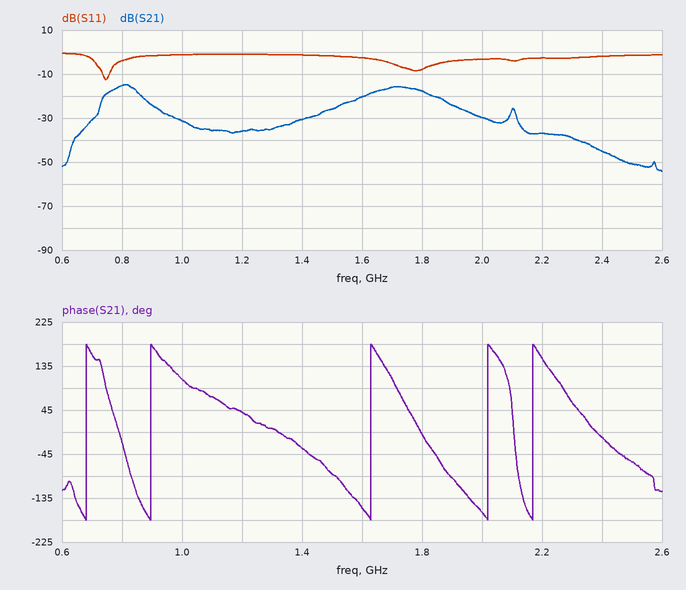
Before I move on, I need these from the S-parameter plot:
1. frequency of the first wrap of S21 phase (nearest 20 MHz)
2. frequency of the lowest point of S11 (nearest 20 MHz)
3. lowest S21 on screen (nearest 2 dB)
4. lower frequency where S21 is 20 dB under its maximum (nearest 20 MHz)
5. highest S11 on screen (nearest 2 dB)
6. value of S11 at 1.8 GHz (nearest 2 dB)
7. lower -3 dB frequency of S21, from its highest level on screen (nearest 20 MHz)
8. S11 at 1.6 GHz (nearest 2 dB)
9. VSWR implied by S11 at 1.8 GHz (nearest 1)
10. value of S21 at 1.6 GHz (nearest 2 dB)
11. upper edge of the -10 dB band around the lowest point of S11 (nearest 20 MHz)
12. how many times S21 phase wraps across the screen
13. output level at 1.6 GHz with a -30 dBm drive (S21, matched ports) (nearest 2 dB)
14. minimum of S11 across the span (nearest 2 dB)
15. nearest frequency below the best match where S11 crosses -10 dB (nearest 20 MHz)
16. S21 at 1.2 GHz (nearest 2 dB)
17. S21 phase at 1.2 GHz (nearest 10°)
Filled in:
680 MHz
740 MHz
-54 dB
680 MHz
0 dB
-8 dB
760 MHz
-2 dB
2
-20 dB
760 MHz
5
-50 dBm
-12 dB
740 MHz
-36 dB
40°
